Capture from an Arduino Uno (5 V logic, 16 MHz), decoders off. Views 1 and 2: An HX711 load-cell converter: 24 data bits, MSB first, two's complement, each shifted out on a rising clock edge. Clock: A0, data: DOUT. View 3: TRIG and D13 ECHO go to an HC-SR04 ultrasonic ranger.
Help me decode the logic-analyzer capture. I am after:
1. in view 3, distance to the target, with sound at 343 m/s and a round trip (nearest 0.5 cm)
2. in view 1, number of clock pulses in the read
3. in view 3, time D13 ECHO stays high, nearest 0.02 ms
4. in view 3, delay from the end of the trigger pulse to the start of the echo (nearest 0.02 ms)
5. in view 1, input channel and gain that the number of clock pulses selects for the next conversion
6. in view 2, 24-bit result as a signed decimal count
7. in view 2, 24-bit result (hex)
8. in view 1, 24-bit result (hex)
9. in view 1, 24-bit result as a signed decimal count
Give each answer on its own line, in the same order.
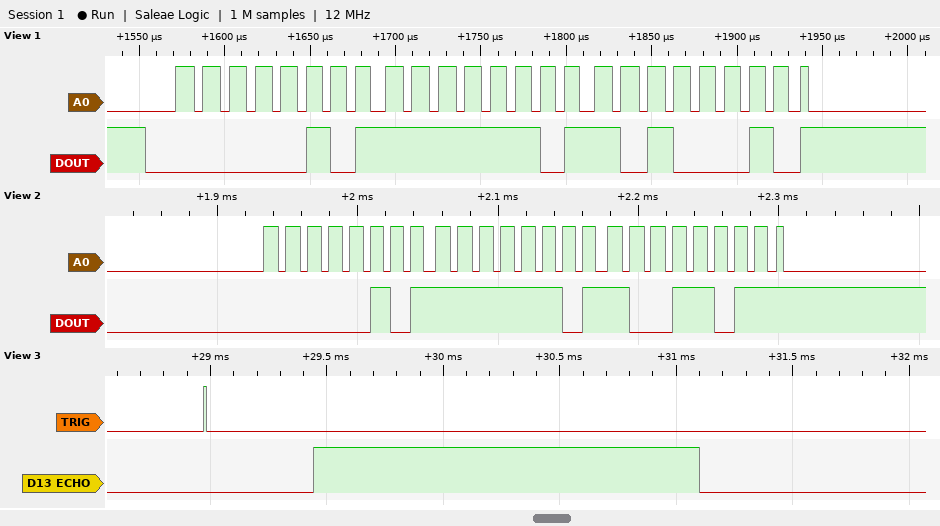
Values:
28.5 cm
25
1.66 ms
0.46 ms
channel A, gain 128
392603
0x05FD9B
0x05FDA2
392610
